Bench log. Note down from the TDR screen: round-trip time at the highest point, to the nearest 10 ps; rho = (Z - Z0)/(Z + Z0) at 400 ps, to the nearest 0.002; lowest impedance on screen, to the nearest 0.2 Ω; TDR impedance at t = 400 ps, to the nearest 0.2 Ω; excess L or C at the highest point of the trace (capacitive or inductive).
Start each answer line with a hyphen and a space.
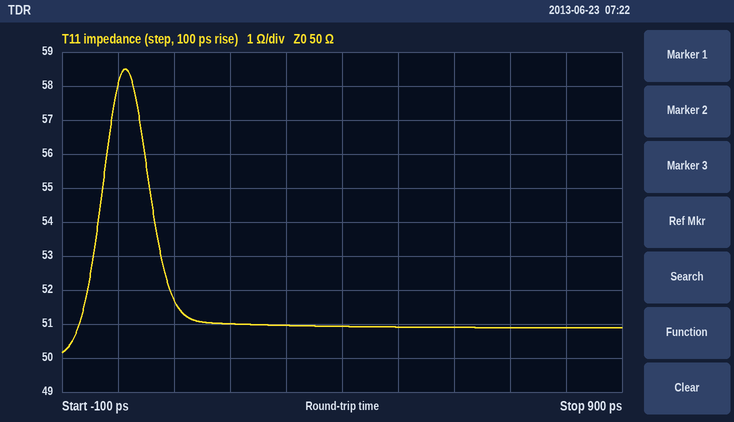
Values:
- 10 ps
- +0.010
- 50.2 Ω
- 51.0 Ω
- inductive
